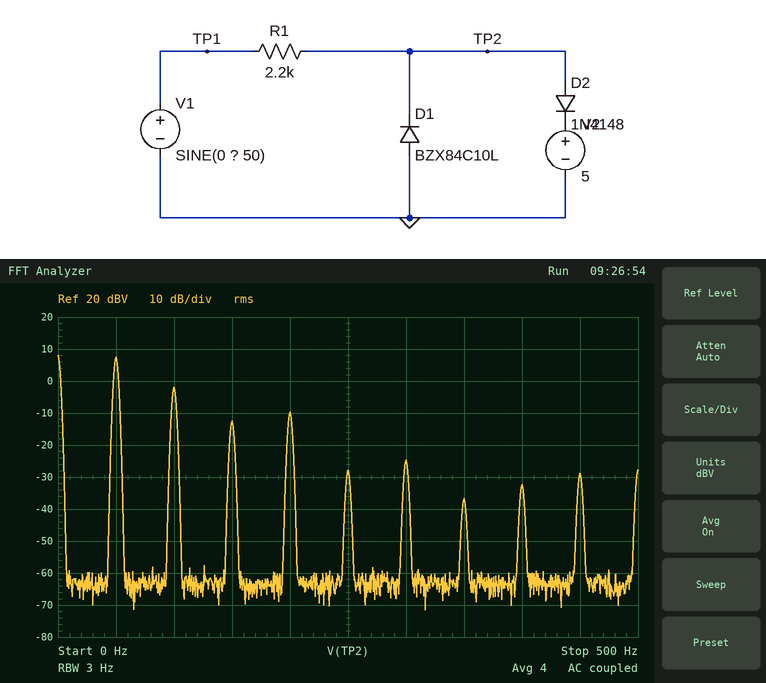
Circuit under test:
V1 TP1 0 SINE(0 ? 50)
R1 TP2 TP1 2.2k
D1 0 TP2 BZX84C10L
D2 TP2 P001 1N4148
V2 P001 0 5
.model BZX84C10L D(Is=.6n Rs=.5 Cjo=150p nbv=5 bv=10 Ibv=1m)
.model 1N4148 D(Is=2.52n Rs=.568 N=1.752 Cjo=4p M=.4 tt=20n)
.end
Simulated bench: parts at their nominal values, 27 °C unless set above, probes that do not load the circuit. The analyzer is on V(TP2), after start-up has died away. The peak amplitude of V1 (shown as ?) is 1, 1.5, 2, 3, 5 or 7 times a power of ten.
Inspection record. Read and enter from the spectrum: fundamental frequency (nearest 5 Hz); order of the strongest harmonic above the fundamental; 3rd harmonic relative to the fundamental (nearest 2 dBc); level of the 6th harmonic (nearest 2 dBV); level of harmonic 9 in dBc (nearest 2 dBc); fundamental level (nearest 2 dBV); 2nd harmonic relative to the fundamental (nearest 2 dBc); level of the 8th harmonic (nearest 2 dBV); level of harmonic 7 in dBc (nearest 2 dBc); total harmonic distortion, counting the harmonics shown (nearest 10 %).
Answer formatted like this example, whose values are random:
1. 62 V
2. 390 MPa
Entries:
1. 50 Hz
2. 2
3. -20 dBc
4. -24 dBV
5. -36 dBc
6. 8 dBV
7. -10 dBc
8. -32 dBV
9. -44 dBc
10. 40 %
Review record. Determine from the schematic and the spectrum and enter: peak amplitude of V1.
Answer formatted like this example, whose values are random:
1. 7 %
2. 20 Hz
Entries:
1. 7 V
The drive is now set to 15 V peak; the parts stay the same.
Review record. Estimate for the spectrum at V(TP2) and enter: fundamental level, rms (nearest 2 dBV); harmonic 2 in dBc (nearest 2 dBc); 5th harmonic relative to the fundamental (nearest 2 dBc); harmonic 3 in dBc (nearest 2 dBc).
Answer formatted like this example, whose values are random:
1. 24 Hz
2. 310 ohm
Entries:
1. 8 dBV
2. -16 dBc
3. -20 dBc
4. -12 dBc
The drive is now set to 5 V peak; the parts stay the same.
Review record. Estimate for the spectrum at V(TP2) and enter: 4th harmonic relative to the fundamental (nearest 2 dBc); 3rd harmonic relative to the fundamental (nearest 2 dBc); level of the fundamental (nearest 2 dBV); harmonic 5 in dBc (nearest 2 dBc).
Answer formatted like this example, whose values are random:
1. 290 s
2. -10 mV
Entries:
1. -22 dBc
2. -32 dBc
3. 6 dBV
4. -36 dBc
